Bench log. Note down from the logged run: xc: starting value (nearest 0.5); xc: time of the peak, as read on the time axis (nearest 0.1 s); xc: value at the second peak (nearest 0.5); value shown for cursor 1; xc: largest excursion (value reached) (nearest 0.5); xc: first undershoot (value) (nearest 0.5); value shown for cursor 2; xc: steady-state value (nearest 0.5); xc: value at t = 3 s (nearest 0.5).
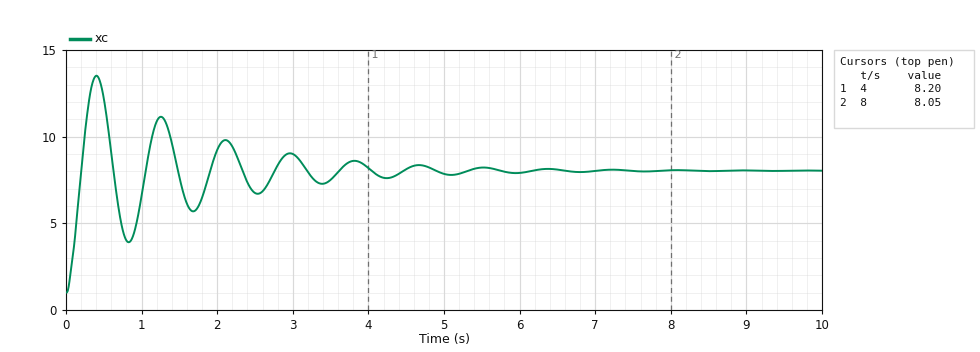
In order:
1.0
0.4 s
11.0
8.20
13.5
4.0
8.05
8.0
9.0
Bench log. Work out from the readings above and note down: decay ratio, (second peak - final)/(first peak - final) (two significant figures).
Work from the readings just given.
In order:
0.55
